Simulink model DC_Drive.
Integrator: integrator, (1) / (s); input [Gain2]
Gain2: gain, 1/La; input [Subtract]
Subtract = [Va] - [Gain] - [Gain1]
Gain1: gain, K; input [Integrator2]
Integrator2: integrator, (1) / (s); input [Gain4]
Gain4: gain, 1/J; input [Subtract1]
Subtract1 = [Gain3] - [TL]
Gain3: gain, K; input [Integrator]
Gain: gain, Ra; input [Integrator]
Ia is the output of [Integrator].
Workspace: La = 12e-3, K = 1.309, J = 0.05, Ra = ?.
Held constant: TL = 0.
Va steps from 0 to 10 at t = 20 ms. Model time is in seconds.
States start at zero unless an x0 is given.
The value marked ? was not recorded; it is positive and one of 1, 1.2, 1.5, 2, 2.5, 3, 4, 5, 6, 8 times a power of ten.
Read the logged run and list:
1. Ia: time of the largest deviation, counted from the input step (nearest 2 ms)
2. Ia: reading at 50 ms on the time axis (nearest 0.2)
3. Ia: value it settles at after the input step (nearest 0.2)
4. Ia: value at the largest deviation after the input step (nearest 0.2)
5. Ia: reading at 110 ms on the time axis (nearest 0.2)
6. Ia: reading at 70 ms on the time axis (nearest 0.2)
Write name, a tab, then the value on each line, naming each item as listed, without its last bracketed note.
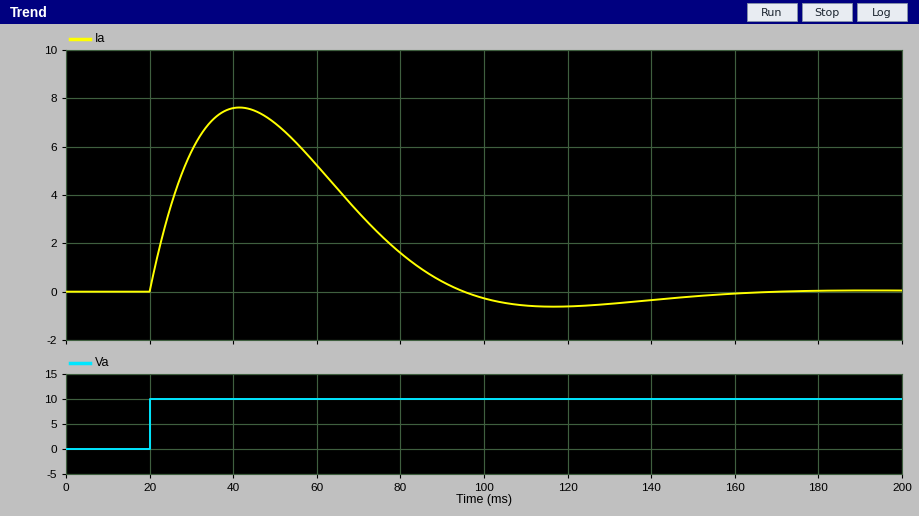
Ia: time of the largest deviation, counted from the input step	22 ms
Ia: reading at 50 ms on the time axis	7.0
Ia: value it settles at after the input step	0.0
Ia: value at the largest deviation after the input step	7.6
Ia: reading at 110 ms on the time axis	-0.6
Ia: reading at 70 ms on the time axis	3.2
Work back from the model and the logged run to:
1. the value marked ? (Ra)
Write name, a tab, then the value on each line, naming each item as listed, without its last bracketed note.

the value marked ?	0.8
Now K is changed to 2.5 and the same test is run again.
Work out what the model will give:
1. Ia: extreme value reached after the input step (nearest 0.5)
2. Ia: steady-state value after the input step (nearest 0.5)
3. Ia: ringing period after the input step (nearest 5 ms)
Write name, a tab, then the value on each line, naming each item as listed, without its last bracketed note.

Ia: extreme value reached after the input step	5.5
Ia: steady-state value after the input step	0.0
Ia: ringing period after the input step	65 ms
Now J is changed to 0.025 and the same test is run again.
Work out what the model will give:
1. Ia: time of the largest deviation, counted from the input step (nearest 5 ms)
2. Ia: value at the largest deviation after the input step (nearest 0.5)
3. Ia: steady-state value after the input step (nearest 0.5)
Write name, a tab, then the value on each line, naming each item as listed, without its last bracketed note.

Ia: time of the largest deviation, counted from the input step	15 ms
Ia: value at the largest deviation after the input step	6.5
Ia: steady-state value after the input step	0.0
